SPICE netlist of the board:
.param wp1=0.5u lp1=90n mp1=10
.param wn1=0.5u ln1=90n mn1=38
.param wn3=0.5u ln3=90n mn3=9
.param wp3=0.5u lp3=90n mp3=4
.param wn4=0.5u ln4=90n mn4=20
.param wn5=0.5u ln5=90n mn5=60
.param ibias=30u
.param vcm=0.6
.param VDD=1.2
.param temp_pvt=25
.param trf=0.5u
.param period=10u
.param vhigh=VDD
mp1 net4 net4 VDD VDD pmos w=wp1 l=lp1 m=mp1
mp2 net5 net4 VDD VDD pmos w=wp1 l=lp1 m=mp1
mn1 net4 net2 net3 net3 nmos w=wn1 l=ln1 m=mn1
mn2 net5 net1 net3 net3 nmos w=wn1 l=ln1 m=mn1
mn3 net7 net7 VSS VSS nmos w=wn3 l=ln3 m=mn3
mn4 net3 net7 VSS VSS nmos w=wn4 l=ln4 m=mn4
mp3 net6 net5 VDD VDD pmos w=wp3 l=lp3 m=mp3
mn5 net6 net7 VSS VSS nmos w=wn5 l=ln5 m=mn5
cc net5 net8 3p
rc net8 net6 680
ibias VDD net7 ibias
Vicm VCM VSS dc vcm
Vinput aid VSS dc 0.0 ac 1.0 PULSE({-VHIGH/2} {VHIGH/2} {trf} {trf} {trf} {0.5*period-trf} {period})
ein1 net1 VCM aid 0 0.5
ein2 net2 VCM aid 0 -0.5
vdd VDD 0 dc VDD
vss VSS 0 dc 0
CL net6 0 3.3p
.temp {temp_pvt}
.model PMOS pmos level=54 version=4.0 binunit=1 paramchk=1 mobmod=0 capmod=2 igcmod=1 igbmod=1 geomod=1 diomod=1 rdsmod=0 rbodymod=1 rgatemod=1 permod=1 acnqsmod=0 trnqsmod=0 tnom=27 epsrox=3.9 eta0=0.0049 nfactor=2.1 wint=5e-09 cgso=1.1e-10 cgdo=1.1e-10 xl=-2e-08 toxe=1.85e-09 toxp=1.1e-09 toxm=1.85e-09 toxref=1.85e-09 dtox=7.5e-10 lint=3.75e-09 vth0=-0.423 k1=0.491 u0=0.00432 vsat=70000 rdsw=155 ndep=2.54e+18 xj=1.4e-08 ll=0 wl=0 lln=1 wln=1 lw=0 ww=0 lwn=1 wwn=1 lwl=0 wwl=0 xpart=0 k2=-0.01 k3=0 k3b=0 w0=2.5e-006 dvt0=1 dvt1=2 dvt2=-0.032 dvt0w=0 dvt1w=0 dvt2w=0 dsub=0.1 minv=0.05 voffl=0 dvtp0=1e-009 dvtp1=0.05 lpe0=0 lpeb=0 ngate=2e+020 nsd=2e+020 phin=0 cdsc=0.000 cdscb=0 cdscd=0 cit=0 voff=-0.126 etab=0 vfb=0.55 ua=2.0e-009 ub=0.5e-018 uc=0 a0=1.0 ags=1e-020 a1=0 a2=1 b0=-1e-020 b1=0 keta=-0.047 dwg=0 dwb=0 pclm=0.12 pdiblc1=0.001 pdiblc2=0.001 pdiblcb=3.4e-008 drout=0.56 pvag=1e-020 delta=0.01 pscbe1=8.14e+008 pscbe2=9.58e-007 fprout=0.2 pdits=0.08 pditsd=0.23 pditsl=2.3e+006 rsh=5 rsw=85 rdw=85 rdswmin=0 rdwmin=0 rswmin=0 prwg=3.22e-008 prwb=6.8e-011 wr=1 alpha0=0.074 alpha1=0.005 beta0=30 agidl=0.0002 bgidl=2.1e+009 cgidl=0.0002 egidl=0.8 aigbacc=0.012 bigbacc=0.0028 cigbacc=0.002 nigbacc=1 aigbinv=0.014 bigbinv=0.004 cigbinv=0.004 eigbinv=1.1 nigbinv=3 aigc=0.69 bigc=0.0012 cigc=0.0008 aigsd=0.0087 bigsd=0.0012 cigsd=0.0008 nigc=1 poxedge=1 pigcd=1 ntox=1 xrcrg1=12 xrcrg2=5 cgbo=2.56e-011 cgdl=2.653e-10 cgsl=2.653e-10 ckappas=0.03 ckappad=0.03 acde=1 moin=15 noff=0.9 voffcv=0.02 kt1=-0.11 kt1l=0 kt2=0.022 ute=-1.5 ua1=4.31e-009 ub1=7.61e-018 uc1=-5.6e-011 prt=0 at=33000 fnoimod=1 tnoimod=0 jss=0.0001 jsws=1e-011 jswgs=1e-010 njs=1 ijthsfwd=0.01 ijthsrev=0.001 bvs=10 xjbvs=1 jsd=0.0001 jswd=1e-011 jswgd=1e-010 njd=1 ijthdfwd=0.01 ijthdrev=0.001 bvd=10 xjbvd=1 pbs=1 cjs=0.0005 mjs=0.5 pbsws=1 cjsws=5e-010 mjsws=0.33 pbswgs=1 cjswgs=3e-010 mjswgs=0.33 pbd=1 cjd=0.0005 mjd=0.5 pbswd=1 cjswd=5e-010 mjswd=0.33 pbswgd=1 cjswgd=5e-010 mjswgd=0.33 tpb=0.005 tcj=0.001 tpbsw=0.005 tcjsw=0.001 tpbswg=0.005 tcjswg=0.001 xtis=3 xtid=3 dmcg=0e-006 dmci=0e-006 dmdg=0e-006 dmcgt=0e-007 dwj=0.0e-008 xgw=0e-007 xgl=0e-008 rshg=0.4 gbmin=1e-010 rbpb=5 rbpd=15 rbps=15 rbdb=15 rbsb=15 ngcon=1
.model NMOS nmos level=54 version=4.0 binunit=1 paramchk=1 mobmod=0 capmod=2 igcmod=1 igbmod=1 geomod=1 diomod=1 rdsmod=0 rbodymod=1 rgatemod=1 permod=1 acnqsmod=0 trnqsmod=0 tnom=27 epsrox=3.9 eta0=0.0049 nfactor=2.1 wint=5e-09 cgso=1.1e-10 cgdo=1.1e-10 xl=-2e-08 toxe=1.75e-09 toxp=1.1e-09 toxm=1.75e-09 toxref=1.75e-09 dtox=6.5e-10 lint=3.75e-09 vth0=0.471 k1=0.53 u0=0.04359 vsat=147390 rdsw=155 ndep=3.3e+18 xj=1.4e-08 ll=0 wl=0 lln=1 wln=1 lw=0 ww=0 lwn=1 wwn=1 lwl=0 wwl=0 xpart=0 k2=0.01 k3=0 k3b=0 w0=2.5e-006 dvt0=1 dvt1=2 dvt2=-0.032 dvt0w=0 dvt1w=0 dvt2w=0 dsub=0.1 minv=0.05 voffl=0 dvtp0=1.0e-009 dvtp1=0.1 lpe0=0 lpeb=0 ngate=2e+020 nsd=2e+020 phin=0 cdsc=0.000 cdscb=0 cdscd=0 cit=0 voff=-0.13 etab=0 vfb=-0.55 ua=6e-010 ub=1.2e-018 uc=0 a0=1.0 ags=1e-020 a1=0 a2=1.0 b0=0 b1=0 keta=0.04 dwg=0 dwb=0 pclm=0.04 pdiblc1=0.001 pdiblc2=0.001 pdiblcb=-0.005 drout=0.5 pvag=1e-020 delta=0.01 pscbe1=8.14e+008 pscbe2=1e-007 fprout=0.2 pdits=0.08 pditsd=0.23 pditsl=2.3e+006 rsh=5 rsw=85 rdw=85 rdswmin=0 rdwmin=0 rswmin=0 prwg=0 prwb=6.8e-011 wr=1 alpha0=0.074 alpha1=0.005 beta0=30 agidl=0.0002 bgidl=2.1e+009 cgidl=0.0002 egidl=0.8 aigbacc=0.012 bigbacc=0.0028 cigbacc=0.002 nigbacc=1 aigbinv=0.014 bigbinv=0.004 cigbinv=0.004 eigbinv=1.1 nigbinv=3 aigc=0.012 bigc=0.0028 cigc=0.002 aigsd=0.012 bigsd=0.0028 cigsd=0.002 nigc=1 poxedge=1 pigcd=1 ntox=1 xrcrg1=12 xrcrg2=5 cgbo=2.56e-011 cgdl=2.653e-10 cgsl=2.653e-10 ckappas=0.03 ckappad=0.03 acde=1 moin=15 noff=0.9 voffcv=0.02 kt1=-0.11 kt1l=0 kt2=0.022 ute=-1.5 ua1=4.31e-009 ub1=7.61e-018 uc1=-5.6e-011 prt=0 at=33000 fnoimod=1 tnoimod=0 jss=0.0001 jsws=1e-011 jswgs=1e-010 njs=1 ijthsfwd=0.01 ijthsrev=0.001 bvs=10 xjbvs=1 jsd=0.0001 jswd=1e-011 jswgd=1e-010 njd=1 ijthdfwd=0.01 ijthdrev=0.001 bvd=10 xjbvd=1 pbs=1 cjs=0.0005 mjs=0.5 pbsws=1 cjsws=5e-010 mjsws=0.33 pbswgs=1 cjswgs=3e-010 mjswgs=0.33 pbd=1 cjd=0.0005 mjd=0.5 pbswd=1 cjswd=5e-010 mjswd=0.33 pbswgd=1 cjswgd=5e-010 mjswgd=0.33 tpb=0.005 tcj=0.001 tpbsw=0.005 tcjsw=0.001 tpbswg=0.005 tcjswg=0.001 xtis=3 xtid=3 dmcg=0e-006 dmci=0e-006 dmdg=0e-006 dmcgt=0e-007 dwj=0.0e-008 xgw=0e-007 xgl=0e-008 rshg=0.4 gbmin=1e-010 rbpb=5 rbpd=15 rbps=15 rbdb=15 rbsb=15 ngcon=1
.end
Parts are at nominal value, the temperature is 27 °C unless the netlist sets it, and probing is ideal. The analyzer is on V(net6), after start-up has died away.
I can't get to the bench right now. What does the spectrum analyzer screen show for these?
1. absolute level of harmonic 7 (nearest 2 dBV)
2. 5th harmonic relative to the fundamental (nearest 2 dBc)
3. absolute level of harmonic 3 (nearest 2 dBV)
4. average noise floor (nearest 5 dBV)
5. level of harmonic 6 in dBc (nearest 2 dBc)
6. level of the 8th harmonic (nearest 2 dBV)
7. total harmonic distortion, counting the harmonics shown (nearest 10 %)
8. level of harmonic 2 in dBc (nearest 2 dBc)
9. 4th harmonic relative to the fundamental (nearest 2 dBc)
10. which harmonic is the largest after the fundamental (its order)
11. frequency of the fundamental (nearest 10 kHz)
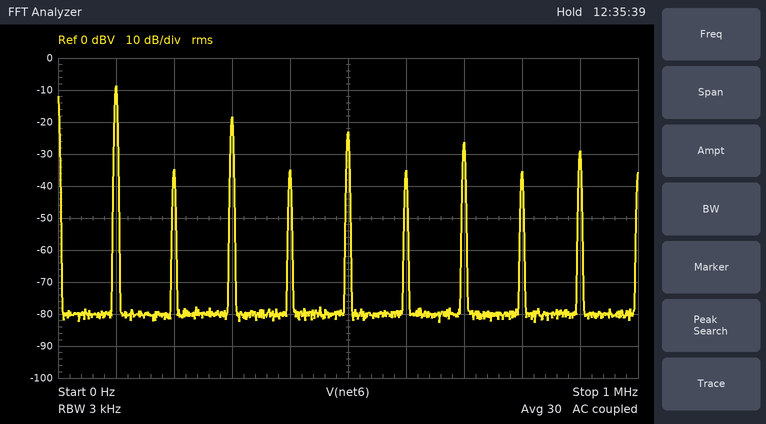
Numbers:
-26 dBV
-14 dBc
-18 dBV
-80 dBV
-26 dBc
-36 dBV
40 %
-26 dBc
-26 dBc
3
100 kHz
